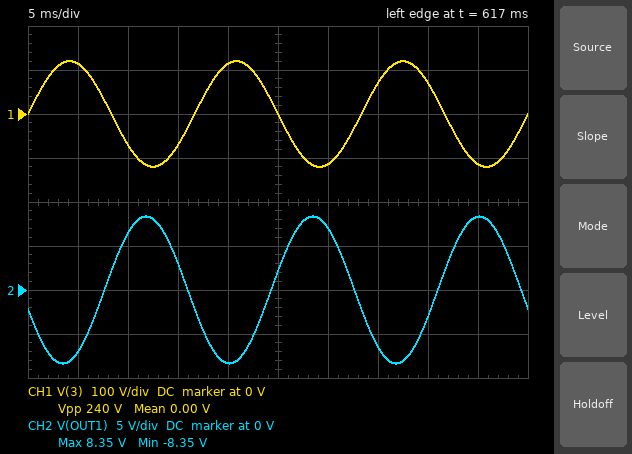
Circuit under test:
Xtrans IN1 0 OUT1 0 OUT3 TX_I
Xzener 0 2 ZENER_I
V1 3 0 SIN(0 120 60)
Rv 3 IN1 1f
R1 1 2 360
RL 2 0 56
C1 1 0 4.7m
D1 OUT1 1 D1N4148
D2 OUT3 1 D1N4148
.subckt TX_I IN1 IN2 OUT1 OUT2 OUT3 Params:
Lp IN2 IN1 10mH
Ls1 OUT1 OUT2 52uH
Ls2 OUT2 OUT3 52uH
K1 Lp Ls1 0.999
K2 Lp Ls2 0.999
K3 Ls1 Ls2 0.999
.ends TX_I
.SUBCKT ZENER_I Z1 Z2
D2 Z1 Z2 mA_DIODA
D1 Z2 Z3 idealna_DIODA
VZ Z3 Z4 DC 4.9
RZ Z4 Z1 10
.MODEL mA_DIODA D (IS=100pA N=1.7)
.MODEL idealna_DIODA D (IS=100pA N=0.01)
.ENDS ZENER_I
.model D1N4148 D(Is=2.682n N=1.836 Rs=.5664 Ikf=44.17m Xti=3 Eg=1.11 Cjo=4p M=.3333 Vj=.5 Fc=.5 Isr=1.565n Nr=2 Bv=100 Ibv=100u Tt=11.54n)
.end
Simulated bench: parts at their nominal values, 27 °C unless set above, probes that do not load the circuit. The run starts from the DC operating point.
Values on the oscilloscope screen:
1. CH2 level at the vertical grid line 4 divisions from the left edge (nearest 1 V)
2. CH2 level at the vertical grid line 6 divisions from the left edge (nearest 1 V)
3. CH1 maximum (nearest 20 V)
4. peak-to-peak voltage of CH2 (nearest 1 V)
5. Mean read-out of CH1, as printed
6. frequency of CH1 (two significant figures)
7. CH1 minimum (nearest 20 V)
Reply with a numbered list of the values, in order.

1. -8 V
2. 7 V
3. 120 V
4. 17 V
5. 0.00 V
6. 60 Hz
7. -120 V
